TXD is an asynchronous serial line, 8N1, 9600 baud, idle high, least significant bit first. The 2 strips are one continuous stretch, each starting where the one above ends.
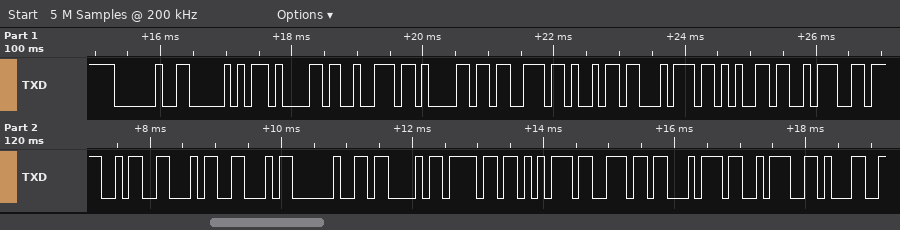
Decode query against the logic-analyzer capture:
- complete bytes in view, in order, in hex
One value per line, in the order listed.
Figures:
20 50 61 72 61 73 69 74 65 3A 4F 46 46 20 43 6F 75 6E 74 3A 31
